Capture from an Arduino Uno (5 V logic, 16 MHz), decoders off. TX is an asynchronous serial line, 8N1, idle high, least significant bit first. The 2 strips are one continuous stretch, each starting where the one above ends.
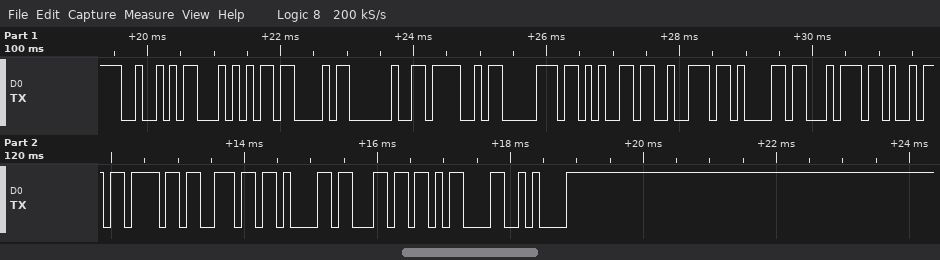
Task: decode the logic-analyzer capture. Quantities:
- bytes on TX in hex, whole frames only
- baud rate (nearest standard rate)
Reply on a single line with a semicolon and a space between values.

0x52 0x54 0x43 0x20 0x4F 0x70 0x65 0x72 0x61 0x74 0x69 0x6F 0x6E 0x61 0x6C 0x0D 0x0A; 9600 baud
